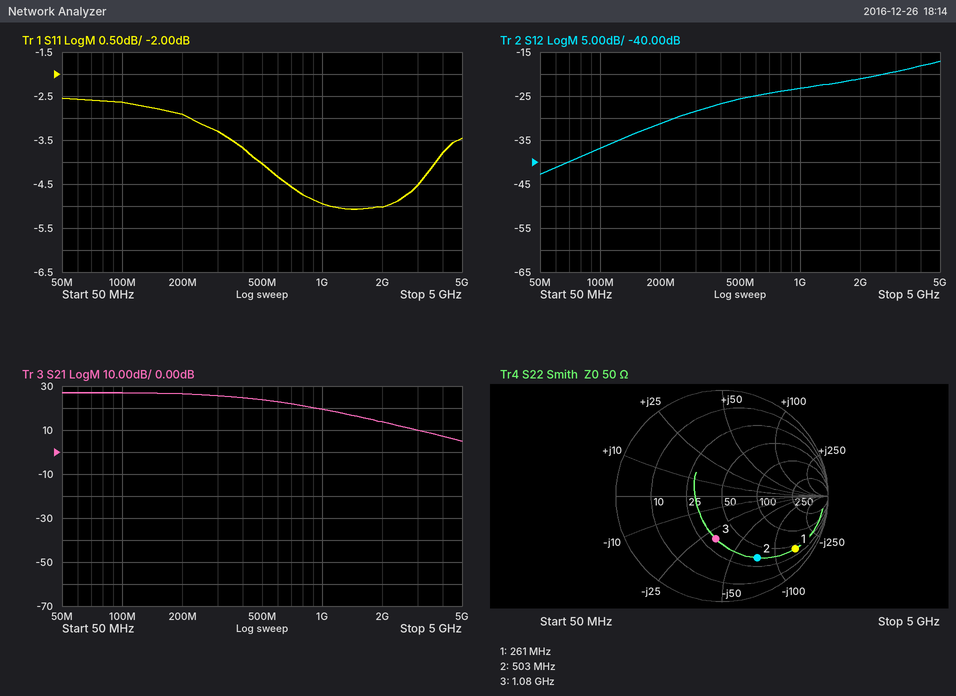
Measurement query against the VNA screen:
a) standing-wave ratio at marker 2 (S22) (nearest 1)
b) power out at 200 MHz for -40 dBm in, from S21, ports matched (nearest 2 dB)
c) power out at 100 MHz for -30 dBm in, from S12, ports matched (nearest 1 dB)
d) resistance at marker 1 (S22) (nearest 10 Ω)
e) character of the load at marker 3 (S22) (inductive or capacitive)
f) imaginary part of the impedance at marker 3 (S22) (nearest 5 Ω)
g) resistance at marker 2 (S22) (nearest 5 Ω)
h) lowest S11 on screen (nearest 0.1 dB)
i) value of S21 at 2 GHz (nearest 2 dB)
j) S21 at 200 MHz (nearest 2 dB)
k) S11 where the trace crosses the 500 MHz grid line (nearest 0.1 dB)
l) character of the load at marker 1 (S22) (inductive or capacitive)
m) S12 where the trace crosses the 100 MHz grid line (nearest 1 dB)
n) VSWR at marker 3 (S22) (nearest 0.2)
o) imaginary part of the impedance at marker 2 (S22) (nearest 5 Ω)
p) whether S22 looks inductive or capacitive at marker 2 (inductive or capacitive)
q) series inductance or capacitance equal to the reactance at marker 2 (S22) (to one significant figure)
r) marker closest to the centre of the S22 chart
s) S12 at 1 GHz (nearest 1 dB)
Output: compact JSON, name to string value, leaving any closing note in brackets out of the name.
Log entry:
{"standing-wave ratio at marker 2 (S22)": "5", "power out at 200 MHz for -40 dBm in, from S21, ports matched": "-14 dBm", "power out at 100 MHz for -30 dBm in, from S12, ports matched": "-67 dBm", "resistance at marker 1 (S22)": "40 Ω", "character of the load at marker 3 (S22)": "capacitive", "imaginary part of the impedance at marker 3 (S22)": "-30 Ω", "resistance at marker 2 (S22)": "35 Ω", "lowest S11 on screen": "-5.1 dB", "value of S21 at 2 GHz": "14 dB", "S21 at 200 MHz": "26 dB", "S11 where the trace crosses the 500 MHz grid line": "-4.0 dB", "character of the load at marker 1 (S22)": "capacitive", "S12 where the trace crosses the 100 MHz grid line": "-37 dB", "VSWR at marker 3 (S22)": "2.4", "imaginary part of the impedance at marker 2 (S22)": "-75 Ω", "whether S22 looks inductive or capacitive at marker 2": "capacitive", "series inductance or capacitance equal to the reactance at marker 2 (S22)": "4 pF", "marker closest to the centre of the S22 chart": "marker 3", "S12 at 1 GHz": "-23 dB"}
